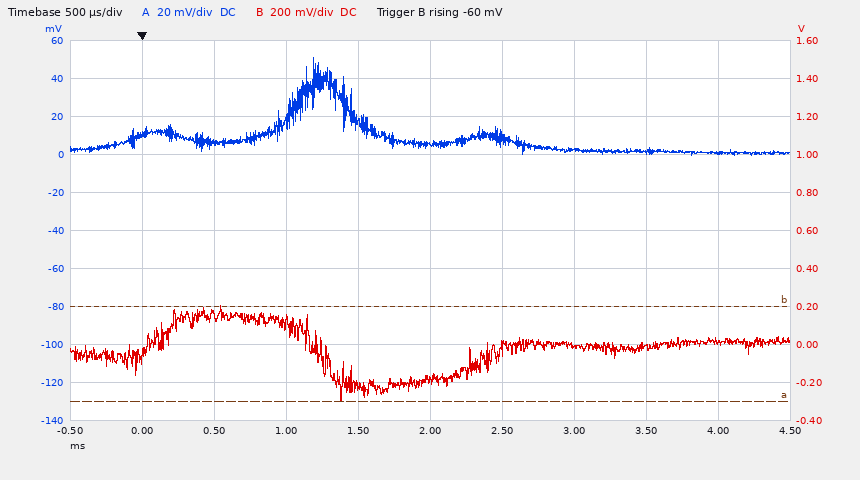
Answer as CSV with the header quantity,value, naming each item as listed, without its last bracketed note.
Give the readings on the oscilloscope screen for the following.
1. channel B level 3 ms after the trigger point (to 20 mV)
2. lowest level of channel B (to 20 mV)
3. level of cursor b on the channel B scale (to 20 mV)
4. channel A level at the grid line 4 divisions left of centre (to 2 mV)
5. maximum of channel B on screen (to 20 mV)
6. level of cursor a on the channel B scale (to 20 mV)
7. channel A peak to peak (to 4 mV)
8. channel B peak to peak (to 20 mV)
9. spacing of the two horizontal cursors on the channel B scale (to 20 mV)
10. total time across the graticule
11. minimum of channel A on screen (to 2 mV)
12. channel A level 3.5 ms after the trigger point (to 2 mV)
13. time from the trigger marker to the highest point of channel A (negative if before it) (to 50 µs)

quantity,value
channel B level 3 ms after the trigger point,0 mV
lowest level of channel B,-300 mV
level of cursor b on the channel B scale,200 mV
channel A level at the grid line 4 divisions left of centre,10 mV
maximum of channel B on screen,200 mV
level of cursor a on the channel B scale,-300 mV
channel A peak to peak,52 mV
channel B peak to peak,500 mV
spacing of the two horizontal cursors on the channel B scale,500 mV
total time across the graticule,5 ms
minimum of channel A on screen,0 mV
channel A level 3.5 ms after the trigger point,2 mV
time from the trigger marker to the highest point of channel A (negative if before it),+1.20 ms
